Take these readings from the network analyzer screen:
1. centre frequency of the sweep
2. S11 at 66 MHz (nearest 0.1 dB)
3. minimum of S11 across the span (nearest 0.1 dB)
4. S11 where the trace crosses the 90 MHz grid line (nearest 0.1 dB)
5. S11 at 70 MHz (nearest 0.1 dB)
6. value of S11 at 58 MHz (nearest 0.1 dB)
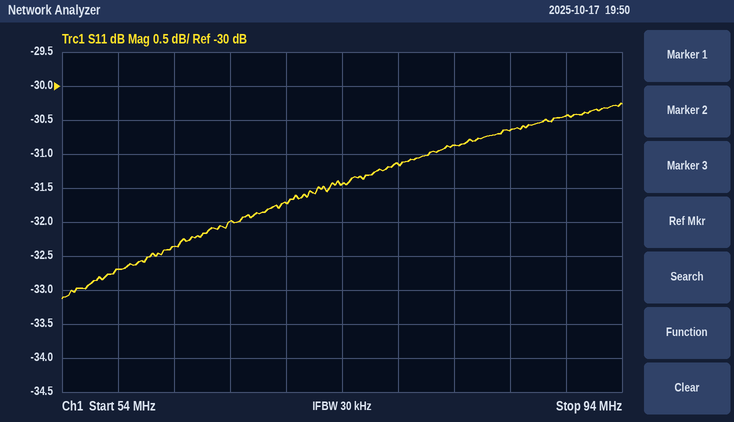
74 MHz
-32.0 dB
-33.1 dB
-30.4 dB
-31.7 dB
-32.7 dB
